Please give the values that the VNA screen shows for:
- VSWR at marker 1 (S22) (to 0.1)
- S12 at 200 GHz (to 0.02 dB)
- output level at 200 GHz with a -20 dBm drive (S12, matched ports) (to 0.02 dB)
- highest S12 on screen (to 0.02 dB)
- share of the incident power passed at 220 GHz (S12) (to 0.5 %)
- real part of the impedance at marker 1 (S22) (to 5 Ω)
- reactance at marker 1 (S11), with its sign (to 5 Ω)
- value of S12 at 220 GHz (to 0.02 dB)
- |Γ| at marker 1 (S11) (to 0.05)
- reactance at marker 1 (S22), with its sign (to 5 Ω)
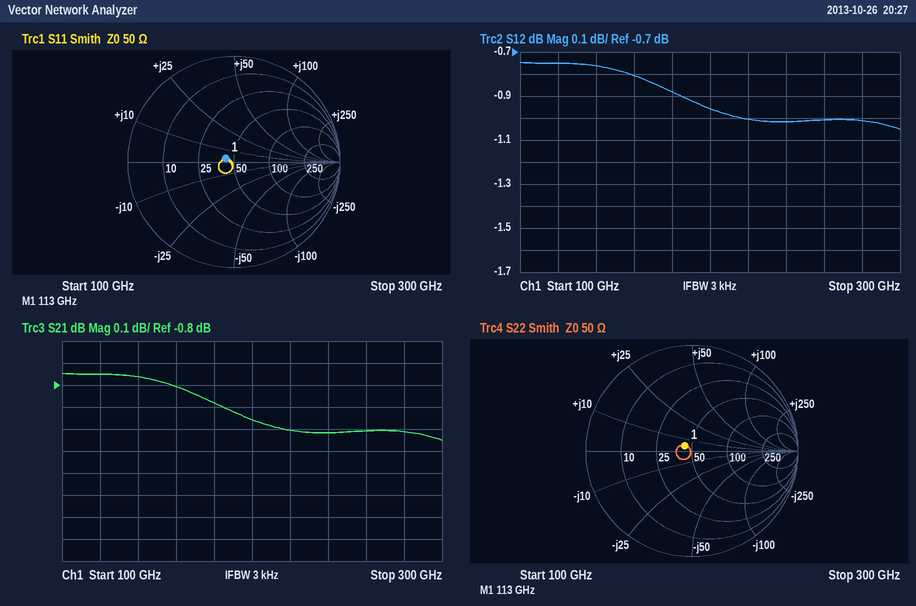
1.2
-0.96 dB
-20.96 dBm
-0.74 dB
79.5 %
45 Ω
+5 Ω
-1.00 dB
0.10
+5 Ω
